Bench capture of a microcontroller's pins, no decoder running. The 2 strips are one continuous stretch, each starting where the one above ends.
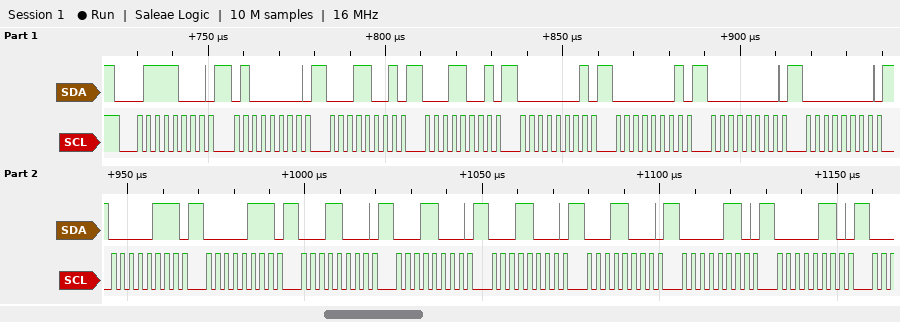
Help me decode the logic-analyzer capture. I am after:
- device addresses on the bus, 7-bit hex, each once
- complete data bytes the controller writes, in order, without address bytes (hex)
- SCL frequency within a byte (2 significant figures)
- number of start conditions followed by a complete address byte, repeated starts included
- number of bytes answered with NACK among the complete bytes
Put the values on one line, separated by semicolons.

0x3C; 40 19 19 01 01 00 00 07 07 18 18 18 18 06 06; 400 kHz; 1; 0
